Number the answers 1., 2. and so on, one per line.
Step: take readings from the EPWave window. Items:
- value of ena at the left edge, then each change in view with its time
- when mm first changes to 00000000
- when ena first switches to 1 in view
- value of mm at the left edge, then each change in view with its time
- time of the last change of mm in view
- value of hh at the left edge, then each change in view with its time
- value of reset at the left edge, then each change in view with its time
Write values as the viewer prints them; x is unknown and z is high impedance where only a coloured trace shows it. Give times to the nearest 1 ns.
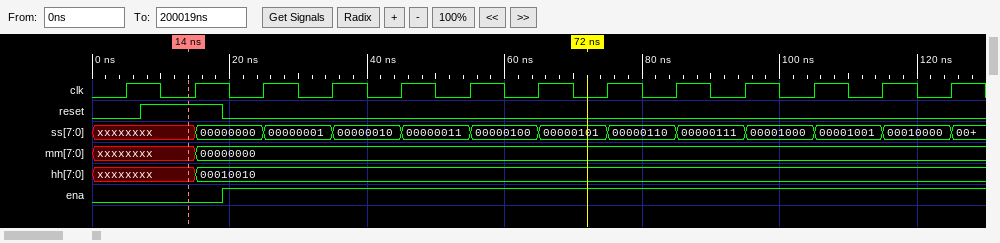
1. 0, 1 at 19 ns
2. 15 ns
3. 19 ns
4. xxxxxxxx, 00000000 at 15 ns
5. 15 ns
6. xxxxxxxx, 00010010 at 15 ns
7. 0, 1 at 7 ns, 0 at 19 ns
